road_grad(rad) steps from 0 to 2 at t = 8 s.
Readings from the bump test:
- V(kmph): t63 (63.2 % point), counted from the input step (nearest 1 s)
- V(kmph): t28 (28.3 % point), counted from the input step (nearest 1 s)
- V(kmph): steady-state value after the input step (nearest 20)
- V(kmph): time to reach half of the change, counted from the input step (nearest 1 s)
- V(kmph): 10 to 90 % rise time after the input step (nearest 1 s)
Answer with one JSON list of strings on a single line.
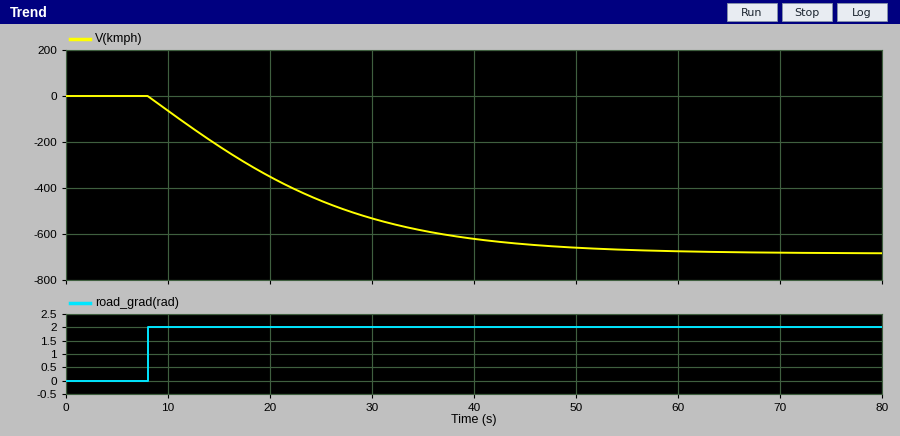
["16 s", "6 s", "-680", "12 s", "29 s"]
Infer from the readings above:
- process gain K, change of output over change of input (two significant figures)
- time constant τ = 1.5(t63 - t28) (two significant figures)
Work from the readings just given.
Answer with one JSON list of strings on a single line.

["-340", "15 s"]
